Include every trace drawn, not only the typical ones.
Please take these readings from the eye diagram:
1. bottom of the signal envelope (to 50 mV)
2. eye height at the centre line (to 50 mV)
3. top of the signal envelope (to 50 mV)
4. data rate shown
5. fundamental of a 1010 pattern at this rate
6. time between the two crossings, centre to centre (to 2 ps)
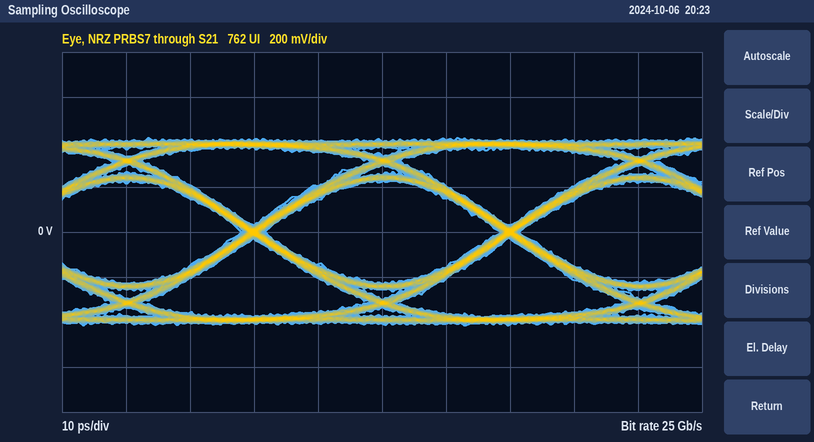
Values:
-400 mV
450 mV
400 mV
25 Gb/s
12.5 GHz
40 ps
